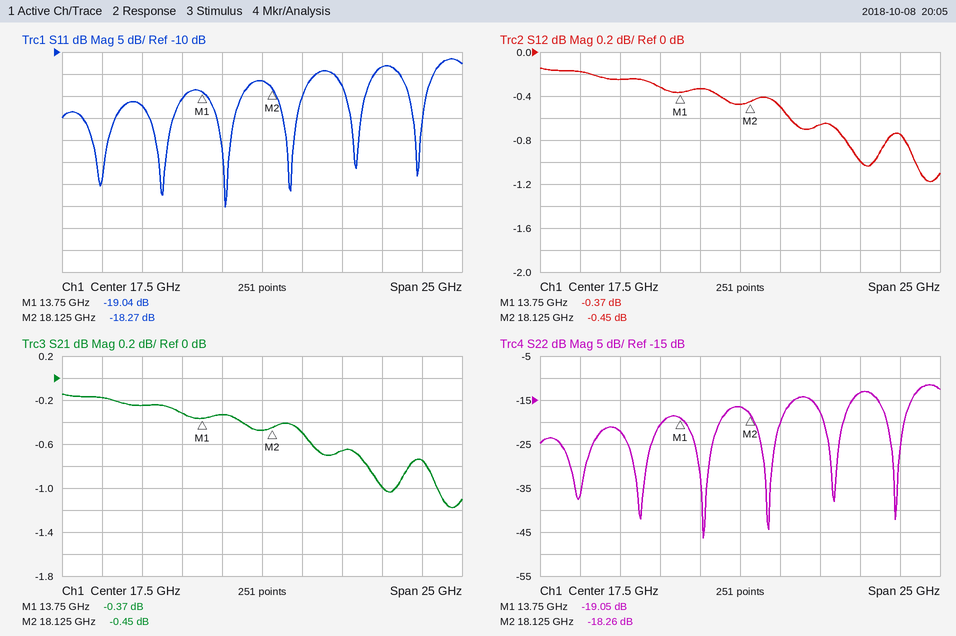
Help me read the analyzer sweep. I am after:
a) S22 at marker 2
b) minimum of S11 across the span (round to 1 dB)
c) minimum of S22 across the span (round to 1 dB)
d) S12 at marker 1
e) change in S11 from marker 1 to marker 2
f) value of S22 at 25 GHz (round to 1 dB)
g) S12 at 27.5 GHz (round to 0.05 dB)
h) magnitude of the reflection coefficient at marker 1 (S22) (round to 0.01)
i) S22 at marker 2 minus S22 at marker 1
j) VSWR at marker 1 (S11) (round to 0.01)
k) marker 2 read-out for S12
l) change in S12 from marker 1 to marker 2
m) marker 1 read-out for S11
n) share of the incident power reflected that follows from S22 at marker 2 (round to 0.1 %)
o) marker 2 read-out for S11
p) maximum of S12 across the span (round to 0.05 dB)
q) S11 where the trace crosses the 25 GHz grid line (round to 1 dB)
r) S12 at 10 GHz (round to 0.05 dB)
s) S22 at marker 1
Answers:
-18.26 dB
-45 dB
-46 dB
-0.37 dB
0.77 dB
-13 dB
-0.75 dB
0.11
0.79 dB
1.25
-0.45 dB
-0.08 dB
-19.04 dB
1.5 %
-18.27 dB
-0.15 dB
-13 dB
-0.25 dB
-19.05 dB
